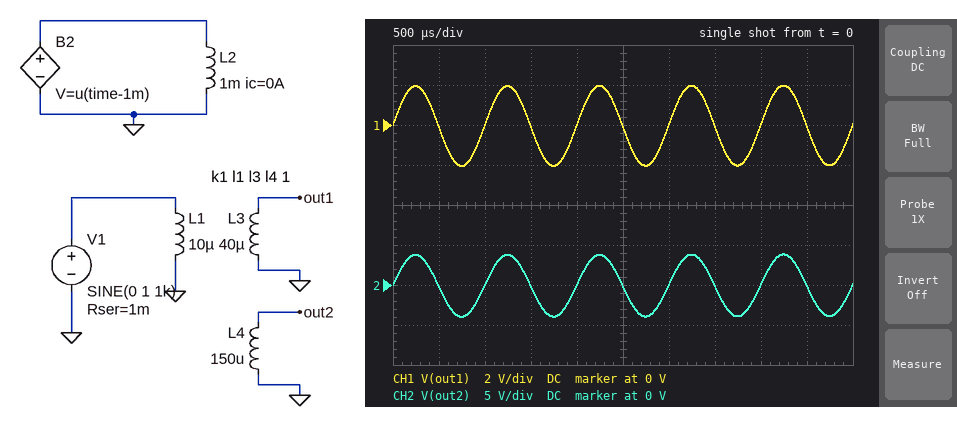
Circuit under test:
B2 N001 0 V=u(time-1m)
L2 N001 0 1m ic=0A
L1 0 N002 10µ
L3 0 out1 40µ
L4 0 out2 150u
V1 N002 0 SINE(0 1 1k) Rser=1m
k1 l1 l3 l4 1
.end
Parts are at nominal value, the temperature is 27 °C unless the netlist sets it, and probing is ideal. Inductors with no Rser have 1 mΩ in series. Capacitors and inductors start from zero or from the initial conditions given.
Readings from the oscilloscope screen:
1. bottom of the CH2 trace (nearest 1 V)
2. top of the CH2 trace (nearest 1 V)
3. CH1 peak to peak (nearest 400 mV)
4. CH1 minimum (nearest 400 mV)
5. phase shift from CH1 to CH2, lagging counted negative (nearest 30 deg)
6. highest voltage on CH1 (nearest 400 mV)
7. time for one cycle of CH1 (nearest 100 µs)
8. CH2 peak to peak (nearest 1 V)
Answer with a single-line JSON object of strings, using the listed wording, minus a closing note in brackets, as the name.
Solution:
{"bottom of the CH2 trace": "-4 V", "top of the CH2 trace": "4 V", "CH1 peak to peak": "4.0 V", "CH1 minimum": "-2.0 V", "phase shift from CH1 to CH2, lagging counted negative": "0 deg", "highest voltage on CH1": "2.0 V", "time for one cycle of CH1": "1.0 ms", "CH2 peak to peak": "8 V"}
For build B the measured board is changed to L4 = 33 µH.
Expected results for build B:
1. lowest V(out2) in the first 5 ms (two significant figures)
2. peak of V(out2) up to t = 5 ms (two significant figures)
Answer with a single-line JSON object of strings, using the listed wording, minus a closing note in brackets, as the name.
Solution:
{"lowest V(out2) in the first 5 ms": "-1.9 V", "peak of V(out2) up to t = 5 ms": "1.8 V"}
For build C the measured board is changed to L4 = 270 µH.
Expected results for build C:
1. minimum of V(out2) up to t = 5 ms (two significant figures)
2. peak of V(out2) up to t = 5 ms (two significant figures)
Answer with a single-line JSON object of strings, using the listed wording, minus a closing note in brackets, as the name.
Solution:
{"minimum of V(out2) up to t = 5 ms": "-5.3 V", "peak of V(out2) up to t = 5 ms": "5.1 V"}
